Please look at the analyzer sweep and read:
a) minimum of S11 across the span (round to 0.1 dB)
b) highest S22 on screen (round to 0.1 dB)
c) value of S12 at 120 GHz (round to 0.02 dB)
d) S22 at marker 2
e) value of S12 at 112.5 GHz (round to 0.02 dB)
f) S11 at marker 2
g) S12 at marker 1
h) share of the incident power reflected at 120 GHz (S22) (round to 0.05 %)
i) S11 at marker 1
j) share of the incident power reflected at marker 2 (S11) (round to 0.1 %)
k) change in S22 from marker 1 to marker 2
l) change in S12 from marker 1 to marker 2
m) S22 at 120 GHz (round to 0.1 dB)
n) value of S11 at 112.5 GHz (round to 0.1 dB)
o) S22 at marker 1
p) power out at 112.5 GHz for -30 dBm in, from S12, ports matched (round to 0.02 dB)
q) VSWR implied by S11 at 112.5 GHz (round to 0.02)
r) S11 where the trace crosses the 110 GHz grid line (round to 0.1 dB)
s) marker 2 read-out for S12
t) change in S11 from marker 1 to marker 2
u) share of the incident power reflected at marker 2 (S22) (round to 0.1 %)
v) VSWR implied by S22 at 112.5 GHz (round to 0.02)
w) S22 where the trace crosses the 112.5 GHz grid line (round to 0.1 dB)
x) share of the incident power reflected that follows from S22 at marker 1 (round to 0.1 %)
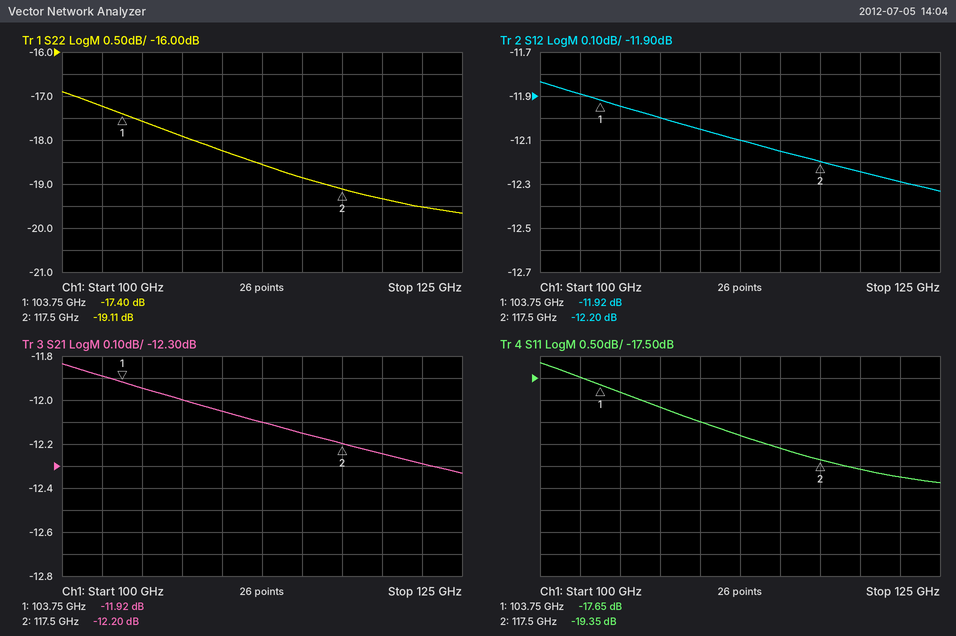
-19.9 dB
-16.9 dB
-12.24 dB
-19.11 dB
-12.10 dB
-19.35 dB
-11.92 dB
1.15 %
-17.65 dB
1.2 %
-1.71 dB
-0.28 dB
-19.3 dB
-18.8 dB
-17.40 dB
-42.10 dBm
1.26
-18.5 dB
-12.20 dB
-1.70 dB
1.2 %
1.26
-18.6 dB
1.8 %
